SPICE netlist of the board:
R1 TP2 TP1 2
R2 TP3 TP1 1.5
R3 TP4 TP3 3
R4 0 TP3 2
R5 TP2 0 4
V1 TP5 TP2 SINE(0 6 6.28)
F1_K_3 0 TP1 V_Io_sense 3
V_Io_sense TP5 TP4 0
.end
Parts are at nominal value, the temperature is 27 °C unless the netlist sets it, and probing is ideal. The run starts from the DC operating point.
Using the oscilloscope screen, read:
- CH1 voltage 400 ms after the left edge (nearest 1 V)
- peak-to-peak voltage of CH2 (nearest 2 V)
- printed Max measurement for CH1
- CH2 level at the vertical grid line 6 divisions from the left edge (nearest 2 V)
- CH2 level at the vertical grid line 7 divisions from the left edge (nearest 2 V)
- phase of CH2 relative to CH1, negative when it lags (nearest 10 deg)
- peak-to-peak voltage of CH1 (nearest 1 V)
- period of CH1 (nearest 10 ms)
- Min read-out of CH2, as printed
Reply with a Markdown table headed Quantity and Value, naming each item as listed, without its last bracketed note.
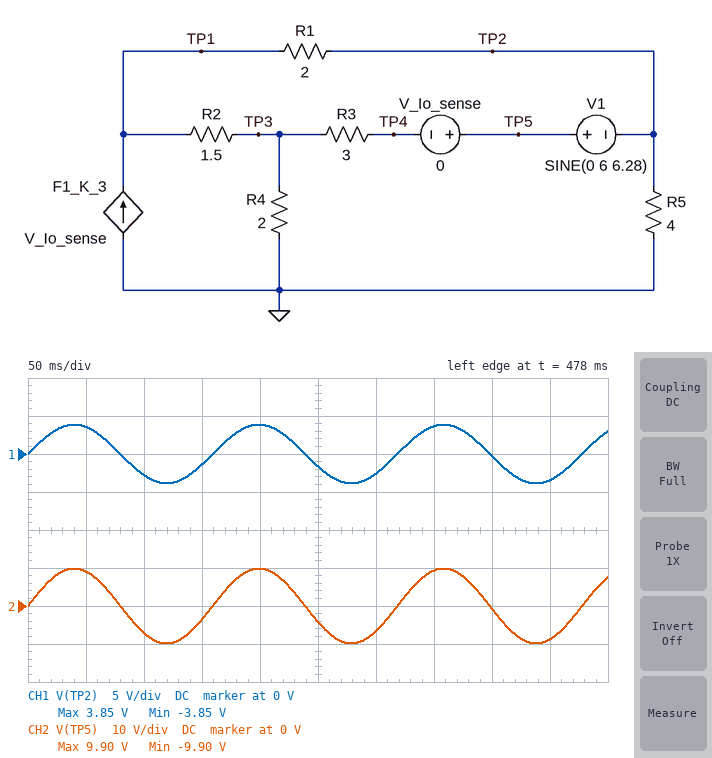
| Quantity | Value |
|---|---|
| CH1 voltage 400 ms after the left edge | 0 V |
| peak-to-peak voltage of CH2 | 20 V |
| printed Max measurement for CH1 | 3.85 V |
| CH2 level at the vertical grid line 6 divisions from the left edge | -6 V |
| CH2 level at the vertical grid line 7 divisions from the left edge | 10 V |
| phase of CH2 relative to CH1, negative when it lags | 0 deg |
| peak-to-peak voltage of CH1 | 8 V |
| period of CH1 | 160 ms |
| Min read-out of CH2, as printed | -9.90 V |
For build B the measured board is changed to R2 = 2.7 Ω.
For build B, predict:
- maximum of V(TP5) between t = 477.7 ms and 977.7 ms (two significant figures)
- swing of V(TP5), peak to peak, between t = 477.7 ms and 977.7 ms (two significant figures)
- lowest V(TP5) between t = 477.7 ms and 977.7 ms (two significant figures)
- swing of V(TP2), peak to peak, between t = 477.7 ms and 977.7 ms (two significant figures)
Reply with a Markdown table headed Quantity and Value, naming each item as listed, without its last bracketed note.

| Quantity | Value |
|---|---|
| maximum of V(TP5) between t = 477.7 ms and 977.7 ms | 12 V |
| swing of V(TP5), peak to peak, between t = 477.7 ms and 977.7 ms | 23 V |
| lowest V(TP5) between t = 477.7 ms and 977.7 ms | -12 V |
| swing of V(TP2), peak to peak, between t = 477.7 ms and 977.7 ms | 11 V |
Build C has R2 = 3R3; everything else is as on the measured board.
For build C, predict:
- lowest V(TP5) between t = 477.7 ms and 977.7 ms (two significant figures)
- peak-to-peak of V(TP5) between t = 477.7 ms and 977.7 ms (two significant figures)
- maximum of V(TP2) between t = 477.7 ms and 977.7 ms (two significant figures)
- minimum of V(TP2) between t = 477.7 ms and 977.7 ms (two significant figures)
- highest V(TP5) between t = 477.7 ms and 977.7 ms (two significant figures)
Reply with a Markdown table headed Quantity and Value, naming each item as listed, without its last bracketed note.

| Quantity | Value |
|---|---|
| lowest V(TP5) between t = 477.7 ms and 977.7 ms | -13 V |
| peak-to-peak of V(TP5) between t = 477.7 ms and 977.7 ms | 25 V |
| maximum of V(TP2) between t = 477.7 ms and 977.7 ms | 6.7 V |
| minimum of V(TP2) between t = 477.7 ms and 977.7 ms | -6.7 V |
| highest V(TP5) between t = 477.7 ms and 977.7 ms | 13 V |
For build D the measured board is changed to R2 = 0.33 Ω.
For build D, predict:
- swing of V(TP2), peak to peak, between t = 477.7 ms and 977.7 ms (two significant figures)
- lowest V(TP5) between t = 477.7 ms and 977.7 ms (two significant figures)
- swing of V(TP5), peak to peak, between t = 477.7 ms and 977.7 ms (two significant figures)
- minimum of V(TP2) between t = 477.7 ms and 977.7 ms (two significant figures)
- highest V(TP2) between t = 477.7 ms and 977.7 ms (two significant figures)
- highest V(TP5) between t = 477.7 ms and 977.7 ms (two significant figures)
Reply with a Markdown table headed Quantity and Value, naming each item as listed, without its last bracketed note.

| Quantity | Value |
|---|---|
| swing of V(TP2), peak to peak, between t = 477.7 ms and 977.7 ms | 4.8 V |
| lowest V(TP5) between t = 477.7 ms and 977.7 ms | -8.4 V |
| swing of V(TP5), peak to peak, between t = 477.7 ms and 977.7 ms | 17 V |
| minimum of V(TP2) between t = 477.7 ms and 977.7 ms | -2.4 V |
| highest V(TP2) between t = 477.7 ms and 977.7 ms | 2.4 V |
| highest V(TP5) between t = 477.7 ms and 977.7 ms | 8.4 V |
